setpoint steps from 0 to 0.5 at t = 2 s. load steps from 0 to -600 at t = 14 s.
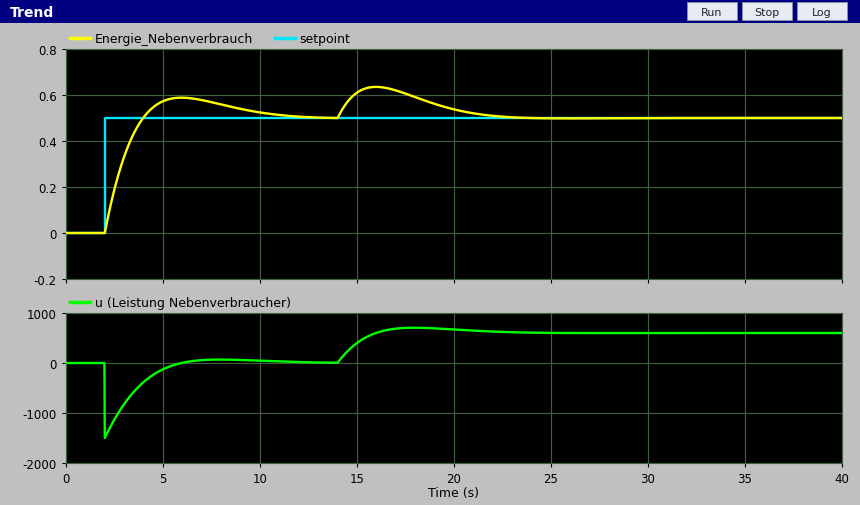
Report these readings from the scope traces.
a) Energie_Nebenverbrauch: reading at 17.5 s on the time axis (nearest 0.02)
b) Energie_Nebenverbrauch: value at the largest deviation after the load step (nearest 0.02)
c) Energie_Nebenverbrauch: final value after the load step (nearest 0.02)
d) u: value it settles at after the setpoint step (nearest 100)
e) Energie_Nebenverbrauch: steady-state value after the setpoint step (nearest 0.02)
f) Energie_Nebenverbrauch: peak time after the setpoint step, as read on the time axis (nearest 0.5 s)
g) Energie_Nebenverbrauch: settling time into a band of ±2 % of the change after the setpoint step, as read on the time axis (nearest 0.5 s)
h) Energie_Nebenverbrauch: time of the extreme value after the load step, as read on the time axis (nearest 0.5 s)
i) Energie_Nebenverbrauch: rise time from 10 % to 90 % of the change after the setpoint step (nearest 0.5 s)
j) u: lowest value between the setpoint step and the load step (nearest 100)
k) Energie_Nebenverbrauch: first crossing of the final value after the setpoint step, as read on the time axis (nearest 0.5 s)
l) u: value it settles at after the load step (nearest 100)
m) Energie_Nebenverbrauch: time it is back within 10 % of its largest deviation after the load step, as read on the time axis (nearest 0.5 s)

0.60
0.64
0.50
0
0.50
6.0 s
11.5 s
16.0 s
1.5 s
-1500
4.0 s
600
21.5 s
